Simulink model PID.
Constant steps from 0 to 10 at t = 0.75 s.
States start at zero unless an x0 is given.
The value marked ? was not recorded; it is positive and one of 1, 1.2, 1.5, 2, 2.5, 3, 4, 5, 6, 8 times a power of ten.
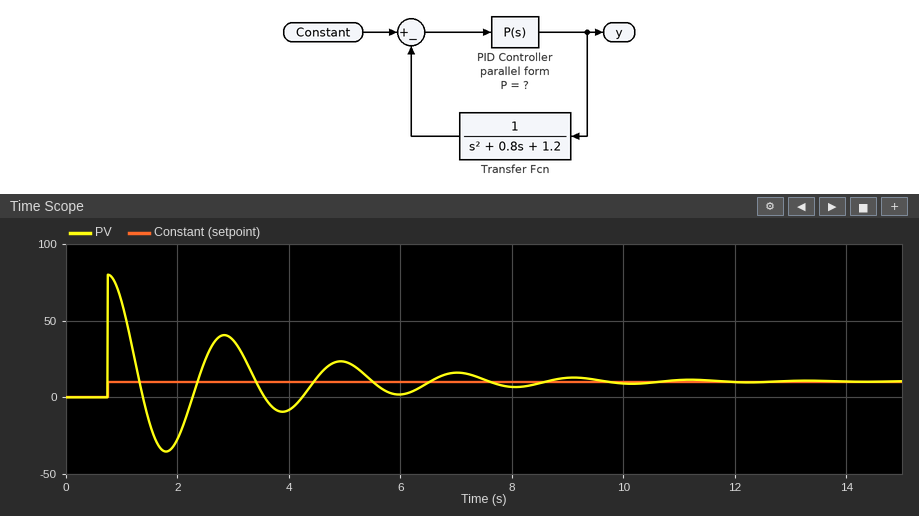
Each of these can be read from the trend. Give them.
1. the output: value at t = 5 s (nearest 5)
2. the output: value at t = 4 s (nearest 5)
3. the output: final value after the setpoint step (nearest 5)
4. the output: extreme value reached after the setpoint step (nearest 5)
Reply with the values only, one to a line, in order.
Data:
25
-10
10
80
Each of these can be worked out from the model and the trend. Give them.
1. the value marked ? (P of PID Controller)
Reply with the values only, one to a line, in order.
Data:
8
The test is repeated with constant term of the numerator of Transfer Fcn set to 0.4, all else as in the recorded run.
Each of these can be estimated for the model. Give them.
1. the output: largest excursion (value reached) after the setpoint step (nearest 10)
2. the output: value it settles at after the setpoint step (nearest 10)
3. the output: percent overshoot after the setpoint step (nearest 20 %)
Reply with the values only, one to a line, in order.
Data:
80
20
260 %
